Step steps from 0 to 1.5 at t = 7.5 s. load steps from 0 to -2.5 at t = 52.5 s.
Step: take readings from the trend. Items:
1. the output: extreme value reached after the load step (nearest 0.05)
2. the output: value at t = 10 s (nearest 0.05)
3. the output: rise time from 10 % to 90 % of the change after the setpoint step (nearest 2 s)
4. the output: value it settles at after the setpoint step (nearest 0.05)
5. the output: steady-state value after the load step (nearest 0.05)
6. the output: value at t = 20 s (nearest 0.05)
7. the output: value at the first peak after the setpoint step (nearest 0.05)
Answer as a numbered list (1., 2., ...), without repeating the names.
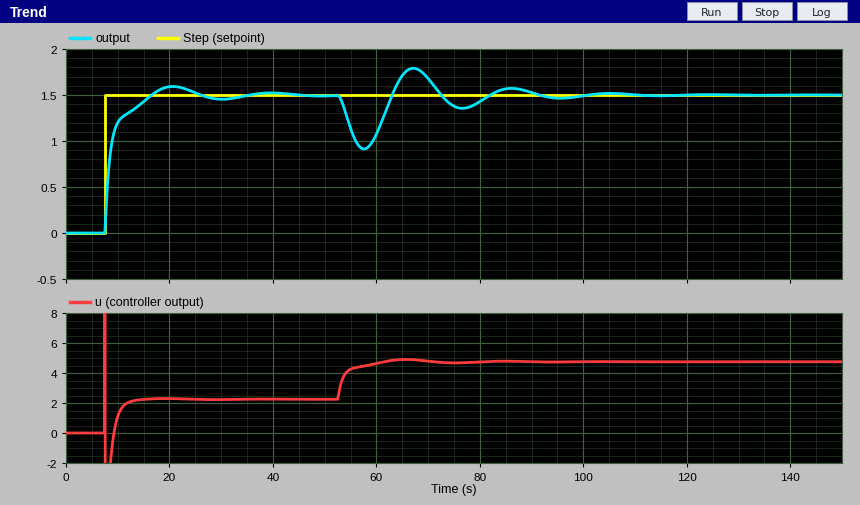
1. 0.90
2. 1.20
3. 6 s
4. 1.50
5. 1.50
6. 1.60
7. 1.60
